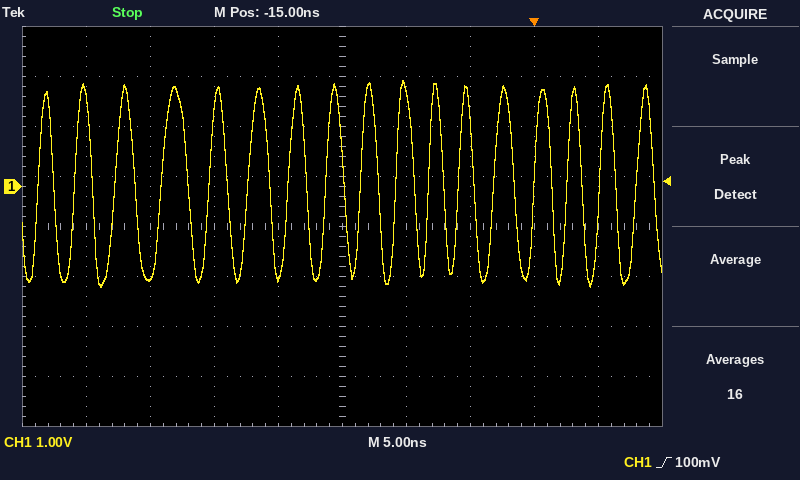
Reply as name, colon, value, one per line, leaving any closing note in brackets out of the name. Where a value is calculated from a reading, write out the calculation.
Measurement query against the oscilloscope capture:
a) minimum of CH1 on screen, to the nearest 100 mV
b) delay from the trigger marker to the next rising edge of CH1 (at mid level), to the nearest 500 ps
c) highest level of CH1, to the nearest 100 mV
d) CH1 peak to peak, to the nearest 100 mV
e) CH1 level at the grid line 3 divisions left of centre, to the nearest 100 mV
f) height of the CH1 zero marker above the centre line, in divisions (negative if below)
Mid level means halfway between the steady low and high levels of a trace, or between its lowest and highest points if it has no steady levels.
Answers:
minimum of CH1 on screen, to the nearest 100 mV: -2.0 V
delay from the trigger marker to the next rising edge of CH1 (at mid level), to the nearest 500 ps: 2.5 ns
highest level of CH1, to the nearest 100 mV: 2.1 V
CH1 peak to peak, to the nearest 100 mV: 2.1 V − (-2.0 V) = 4.1 V
CH1 level at the grid line 3 divisions left of centre, to the nearest 100 mV: -1.8 V
height of the CH1 zero marker above the centre line, in divisions: +0.8 div
